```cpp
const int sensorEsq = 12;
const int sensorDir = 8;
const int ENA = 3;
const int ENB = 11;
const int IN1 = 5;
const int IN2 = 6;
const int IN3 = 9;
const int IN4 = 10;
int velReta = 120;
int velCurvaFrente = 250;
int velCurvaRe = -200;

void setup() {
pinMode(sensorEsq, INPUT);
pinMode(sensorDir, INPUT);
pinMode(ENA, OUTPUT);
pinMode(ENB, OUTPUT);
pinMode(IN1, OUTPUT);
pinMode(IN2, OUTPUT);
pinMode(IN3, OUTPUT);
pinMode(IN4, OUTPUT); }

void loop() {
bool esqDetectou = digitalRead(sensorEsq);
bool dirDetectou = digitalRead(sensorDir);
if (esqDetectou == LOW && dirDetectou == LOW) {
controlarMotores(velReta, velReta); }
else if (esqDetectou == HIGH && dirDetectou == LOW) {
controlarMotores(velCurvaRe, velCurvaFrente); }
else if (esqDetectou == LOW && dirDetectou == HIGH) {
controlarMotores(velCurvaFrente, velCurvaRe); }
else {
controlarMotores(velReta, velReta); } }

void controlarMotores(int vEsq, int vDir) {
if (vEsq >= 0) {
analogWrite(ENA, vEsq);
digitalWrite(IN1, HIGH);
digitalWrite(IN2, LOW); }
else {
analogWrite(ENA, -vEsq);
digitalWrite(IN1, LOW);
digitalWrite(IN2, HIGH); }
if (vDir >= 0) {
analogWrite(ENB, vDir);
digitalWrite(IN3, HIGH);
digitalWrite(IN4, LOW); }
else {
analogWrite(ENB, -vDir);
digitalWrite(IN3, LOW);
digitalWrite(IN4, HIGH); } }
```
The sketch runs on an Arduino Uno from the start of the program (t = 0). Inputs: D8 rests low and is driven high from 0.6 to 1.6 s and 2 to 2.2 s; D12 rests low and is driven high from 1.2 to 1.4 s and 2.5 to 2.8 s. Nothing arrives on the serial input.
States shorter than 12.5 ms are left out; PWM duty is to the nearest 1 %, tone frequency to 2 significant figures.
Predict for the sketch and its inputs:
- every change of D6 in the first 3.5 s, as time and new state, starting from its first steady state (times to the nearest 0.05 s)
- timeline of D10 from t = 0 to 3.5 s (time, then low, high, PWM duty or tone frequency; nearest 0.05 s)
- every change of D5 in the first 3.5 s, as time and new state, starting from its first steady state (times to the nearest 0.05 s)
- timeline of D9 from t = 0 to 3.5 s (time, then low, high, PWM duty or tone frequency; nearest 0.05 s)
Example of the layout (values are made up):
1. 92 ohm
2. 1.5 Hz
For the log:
1. 0 s low; 2.5 s high; 2.8 s low
2. 0 s low; 0.6 s high; 1.2 s low; 1.4 s high; 1.6 s low; 2 s high; 2.2 s low
3. 0 s high; 2.5 s low; 2.8 s high
4. 0 s high; 0.6 s low; 1.2 s high; 1.4 s low; 1.6 s high; 2 s low; 2.2 s high
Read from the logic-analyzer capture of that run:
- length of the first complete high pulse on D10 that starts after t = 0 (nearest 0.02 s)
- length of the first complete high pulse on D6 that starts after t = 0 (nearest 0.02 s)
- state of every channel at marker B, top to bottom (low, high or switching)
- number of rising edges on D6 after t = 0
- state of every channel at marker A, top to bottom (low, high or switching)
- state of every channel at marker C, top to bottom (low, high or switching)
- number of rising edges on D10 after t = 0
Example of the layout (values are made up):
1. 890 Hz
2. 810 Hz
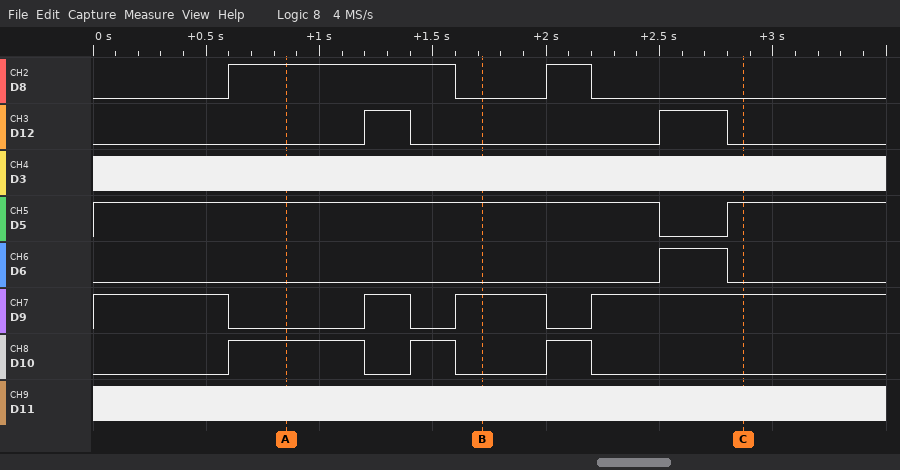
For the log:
1. 0.60 s
2. 0.30 s
3. D8 low, D12 low, D3 switching, D5 high, D6 low, D9 high, D10 low, D11 switching
4. 1
5. D8 high, D12 low, D3 switching, D5 high, D6 low, D9 low, D10 high, D11 switching
6. D8 low, D12 low, D3 switching, D5 high, D6 low, D9 high, D10 low, D11 switching
7. 3
